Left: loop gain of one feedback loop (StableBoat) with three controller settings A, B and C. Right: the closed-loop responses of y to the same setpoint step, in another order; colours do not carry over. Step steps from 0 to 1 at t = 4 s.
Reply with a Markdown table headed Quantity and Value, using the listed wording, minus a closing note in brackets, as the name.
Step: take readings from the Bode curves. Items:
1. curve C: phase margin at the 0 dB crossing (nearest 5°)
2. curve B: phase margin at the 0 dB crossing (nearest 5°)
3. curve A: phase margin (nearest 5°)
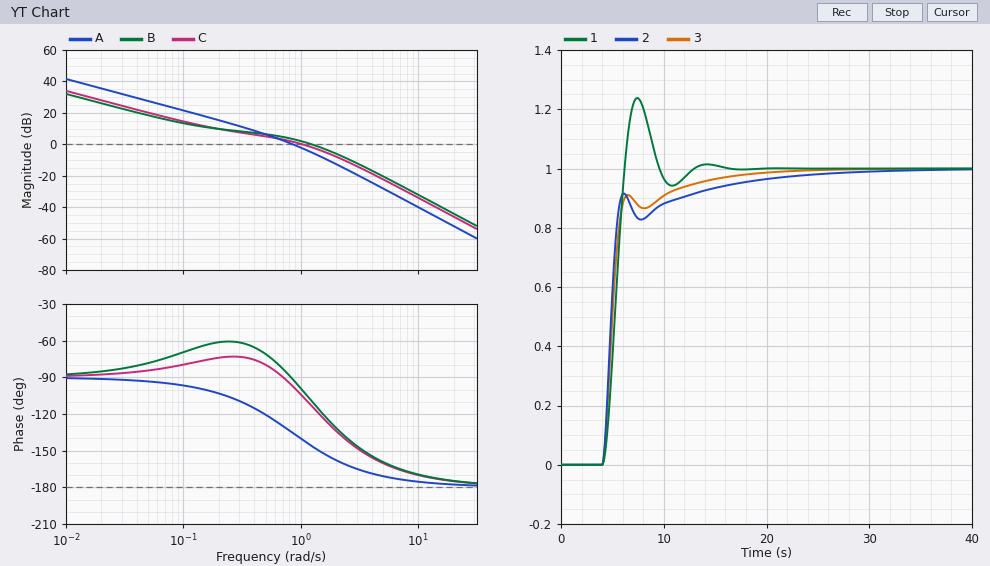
| Quantity | Value |
|---|---|
| curve C: phase margin at the 0 dB crossing | 75° |
| curve B: phase margin at the 0 dB crossing | 70° |
| curve A: phase margin | 45° |
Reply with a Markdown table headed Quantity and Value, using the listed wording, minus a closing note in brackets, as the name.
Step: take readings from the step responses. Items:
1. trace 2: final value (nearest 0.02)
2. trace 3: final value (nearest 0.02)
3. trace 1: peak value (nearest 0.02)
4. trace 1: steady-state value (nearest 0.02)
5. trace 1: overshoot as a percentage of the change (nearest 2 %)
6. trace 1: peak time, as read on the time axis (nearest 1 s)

| Quantity | Value |
|---|---|
| trace 2: final value | 1.00 |
| trace 3: final value | 1.00 |
| trace 1: peak value | 1.24 |
| trace 1: steady-state value | 1.00 |
| trace 1: overshoot as a percentage of the change | 24 % |
| trace 1: peak time, as read on the time axis | 7 s |
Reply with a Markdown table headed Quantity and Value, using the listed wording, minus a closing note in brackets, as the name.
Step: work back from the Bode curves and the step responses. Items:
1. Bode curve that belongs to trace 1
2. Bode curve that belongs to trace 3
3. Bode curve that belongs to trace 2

| Quantity | Value |
|---|---|
| Bode curve that belongs to trace 1 | A |
| Bode curve that belongs to trace 3 | C |
| Bode curve that belongs to trace 2 | B |
